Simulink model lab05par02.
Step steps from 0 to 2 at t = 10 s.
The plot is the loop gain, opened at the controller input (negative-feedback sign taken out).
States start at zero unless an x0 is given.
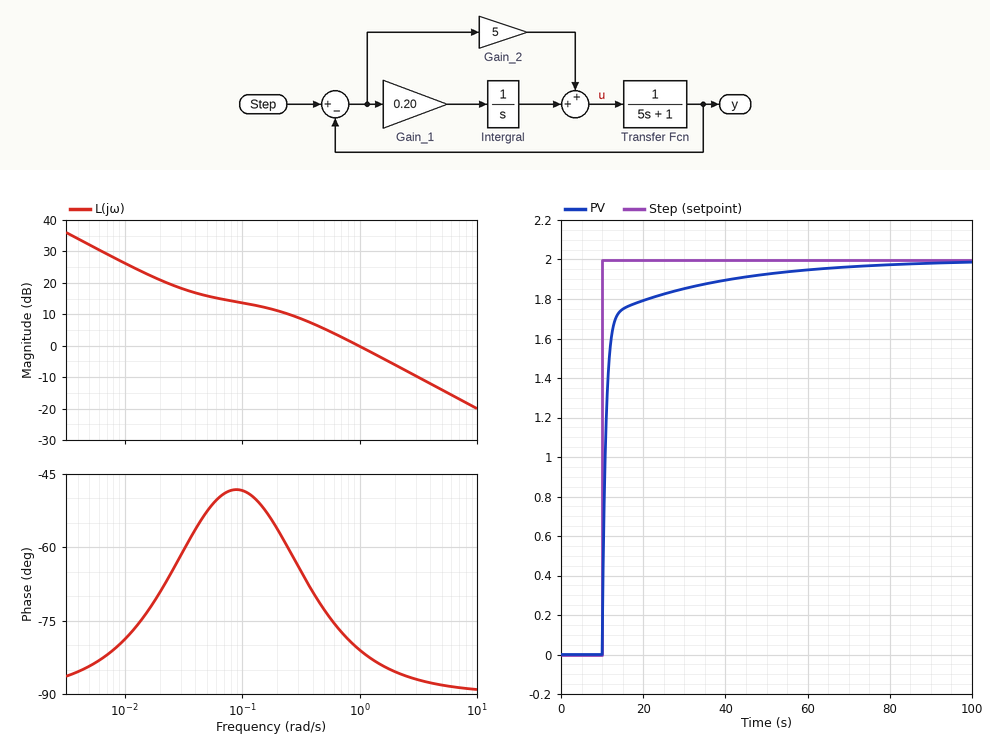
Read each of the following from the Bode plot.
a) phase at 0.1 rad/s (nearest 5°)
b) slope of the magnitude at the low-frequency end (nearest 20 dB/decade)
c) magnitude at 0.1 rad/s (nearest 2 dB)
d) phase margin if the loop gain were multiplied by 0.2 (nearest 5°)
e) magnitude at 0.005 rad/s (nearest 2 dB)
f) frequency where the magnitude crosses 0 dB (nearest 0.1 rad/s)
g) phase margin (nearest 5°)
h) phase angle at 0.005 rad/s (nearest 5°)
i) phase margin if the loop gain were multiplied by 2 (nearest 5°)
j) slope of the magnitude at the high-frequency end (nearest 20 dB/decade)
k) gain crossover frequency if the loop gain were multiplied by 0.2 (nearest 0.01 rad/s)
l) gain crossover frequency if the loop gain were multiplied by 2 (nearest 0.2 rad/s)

-50°
-20 dB/decade
14 dB
130°
32 dB
1.0 rad/s
100°
-85°
95°
-20 dB/decade
0.09 rad/s
2.0 rad/s
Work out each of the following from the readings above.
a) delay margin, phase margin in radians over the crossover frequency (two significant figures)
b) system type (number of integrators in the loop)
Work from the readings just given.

1.7 s
1
